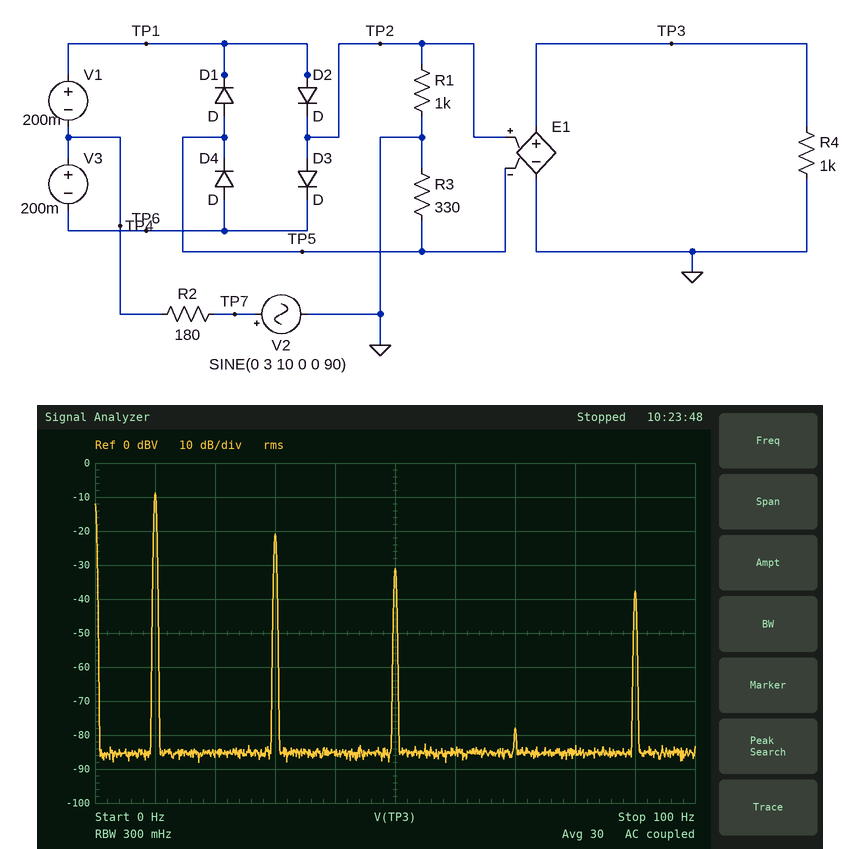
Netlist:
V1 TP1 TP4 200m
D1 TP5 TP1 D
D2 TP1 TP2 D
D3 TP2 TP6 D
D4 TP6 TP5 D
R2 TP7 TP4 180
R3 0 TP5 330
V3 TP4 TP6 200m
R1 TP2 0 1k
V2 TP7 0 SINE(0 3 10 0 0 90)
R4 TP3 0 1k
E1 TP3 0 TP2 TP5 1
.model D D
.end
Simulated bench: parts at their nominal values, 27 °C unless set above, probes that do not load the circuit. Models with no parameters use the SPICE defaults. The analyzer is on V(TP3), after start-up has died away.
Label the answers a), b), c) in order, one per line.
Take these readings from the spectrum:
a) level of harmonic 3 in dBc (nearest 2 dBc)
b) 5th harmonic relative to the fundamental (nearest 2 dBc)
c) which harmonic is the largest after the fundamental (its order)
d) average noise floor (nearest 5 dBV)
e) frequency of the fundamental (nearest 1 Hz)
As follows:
a) -12 dBc
b) -22 dBc
c) 3
d) -85 dBV
e) 10 Hz
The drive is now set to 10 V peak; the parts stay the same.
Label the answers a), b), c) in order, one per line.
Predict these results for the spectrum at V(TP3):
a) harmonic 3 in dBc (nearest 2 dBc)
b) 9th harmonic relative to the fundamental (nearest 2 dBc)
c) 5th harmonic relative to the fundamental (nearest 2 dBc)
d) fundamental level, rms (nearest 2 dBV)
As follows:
a) -10 dBc
b) -22 dBc
c) -14 dBc
d) -8 dBV
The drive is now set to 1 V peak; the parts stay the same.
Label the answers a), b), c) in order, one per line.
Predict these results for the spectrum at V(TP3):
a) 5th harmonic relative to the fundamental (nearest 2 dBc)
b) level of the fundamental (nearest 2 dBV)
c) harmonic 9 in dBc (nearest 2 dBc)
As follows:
a) -18 dBc
b) -12 dBV
c) -38 dBc
